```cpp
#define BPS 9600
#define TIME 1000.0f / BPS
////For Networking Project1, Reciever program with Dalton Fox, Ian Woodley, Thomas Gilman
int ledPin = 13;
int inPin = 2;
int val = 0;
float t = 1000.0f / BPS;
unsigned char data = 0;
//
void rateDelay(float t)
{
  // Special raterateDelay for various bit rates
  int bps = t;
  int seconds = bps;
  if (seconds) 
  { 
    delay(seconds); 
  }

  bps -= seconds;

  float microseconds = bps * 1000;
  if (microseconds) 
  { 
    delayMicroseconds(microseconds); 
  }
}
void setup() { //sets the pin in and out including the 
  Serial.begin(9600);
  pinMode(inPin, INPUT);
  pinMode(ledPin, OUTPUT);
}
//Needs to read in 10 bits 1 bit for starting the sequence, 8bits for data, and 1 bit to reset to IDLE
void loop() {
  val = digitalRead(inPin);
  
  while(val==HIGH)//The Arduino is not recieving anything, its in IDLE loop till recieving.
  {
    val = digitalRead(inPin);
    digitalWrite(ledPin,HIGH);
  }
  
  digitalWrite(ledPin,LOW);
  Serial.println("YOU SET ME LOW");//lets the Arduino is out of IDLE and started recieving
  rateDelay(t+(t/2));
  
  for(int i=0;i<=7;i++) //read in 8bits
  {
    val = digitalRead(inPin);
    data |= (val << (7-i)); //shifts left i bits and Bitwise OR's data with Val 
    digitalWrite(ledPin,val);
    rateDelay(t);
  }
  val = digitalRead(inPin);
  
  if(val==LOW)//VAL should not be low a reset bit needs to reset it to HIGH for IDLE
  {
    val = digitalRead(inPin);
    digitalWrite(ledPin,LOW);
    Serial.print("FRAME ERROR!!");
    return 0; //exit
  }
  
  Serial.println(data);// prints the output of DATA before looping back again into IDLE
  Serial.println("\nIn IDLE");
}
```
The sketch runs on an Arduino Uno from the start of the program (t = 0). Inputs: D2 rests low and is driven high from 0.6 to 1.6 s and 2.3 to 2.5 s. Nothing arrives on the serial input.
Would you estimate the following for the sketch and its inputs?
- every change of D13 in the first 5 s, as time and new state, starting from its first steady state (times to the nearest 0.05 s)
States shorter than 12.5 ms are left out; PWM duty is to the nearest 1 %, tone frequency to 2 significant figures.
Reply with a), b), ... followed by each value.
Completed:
a) 0 s low; 0.6 s high; 1.6 s low; 2.3 s high; 2.5 s low
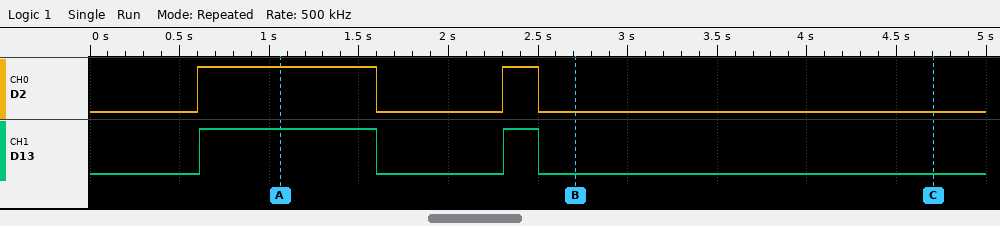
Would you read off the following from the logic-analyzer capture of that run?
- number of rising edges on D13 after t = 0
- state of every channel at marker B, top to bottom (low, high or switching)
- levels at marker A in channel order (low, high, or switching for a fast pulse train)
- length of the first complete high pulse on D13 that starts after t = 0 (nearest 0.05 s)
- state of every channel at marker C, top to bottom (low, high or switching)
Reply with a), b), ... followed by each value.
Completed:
a) 2
b) D2 low, D13 low
c) D2 high, D13 high
d) 1.00 s
e) D2 low, D13 low
